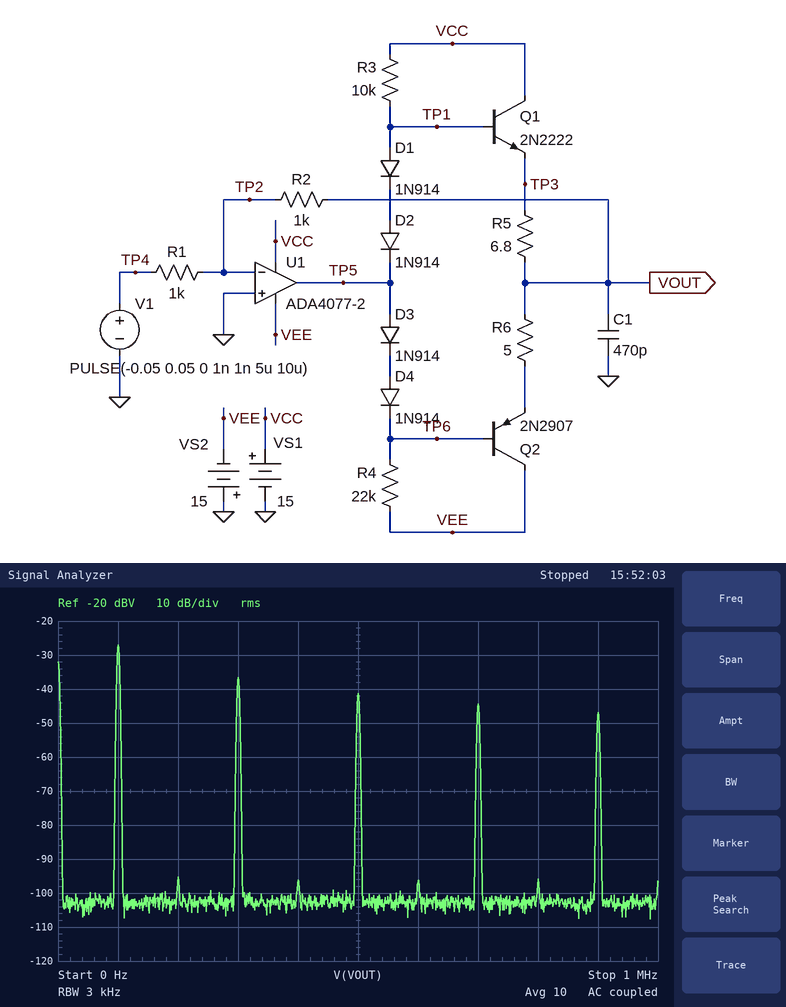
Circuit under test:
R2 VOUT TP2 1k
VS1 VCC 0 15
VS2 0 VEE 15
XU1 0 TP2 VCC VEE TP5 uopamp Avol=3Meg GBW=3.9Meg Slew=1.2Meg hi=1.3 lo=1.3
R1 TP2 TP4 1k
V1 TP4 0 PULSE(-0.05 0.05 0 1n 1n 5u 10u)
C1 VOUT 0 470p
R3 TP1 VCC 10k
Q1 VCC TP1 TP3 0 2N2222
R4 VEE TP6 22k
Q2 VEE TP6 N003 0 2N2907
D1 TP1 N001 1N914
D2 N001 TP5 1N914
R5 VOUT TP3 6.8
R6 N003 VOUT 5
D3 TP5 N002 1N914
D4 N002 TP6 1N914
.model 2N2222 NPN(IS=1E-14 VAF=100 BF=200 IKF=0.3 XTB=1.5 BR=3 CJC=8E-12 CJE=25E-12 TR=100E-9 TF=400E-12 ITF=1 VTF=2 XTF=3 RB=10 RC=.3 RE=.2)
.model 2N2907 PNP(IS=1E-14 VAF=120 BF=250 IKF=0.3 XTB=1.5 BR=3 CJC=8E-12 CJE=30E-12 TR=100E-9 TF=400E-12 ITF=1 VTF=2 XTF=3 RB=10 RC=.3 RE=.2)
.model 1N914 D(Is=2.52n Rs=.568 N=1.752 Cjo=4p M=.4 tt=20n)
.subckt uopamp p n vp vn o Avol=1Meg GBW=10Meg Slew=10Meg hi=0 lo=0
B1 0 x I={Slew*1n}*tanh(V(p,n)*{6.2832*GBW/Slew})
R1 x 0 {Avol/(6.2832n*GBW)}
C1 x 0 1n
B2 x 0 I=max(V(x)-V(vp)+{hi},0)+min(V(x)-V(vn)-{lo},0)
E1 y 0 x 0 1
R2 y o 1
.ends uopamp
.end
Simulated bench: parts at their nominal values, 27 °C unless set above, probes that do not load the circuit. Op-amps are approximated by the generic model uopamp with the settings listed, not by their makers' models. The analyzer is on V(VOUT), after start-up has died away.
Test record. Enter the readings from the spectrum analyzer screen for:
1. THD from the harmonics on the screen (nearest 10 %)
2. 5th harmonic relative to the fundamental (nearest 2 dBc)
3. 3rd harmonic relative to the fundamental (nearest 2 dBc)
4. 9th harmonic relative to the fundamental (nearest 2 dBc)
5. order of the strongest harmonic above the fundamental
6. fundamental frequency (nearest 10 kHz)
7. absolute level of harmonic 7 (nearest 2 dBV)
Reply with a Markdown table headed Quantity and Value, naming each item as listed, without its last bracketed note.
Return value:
| Quantity | Value |
|---|---|
| THD from the harmonics on the screen | 40 % |
| 5th harmonic relative to the fundamental | -14 dBc |
| 3rd harmonic relative to the fundamental | -10 dBc |
| 9th harmonic relative to the fundamental | -20 dBc |
| order of the strongest harmonic above the fundamental | 3 |
| fundamental frequency | 100 kHz |
| absolute level of harmonic 7 | -44 dBV |
